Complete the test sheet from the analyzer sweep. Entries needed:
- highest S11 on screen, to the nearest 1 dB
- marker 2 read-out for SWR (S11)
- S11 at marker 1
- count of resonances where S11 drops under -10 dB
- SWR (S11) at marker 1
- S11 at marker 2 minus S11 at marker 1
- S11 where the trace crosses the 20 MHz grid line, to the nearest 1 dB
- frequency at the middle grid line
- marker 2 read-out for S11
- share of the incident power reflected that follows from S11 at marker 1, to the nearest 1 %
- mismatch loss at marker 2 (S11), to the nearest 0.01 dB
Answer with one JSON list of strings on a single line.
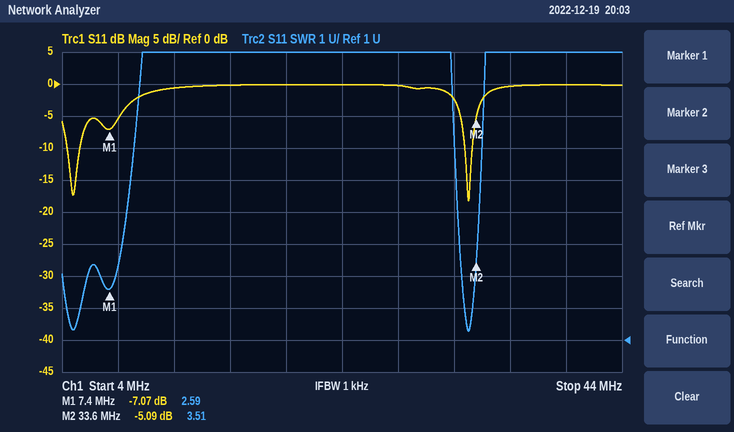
["0 dB", "3.51", "-7.07 dB", "2", "2.59", "1.98 dB", "0 dB", "24 MHz", "-5.09 dB", "20 %", "1.61 dB"]
